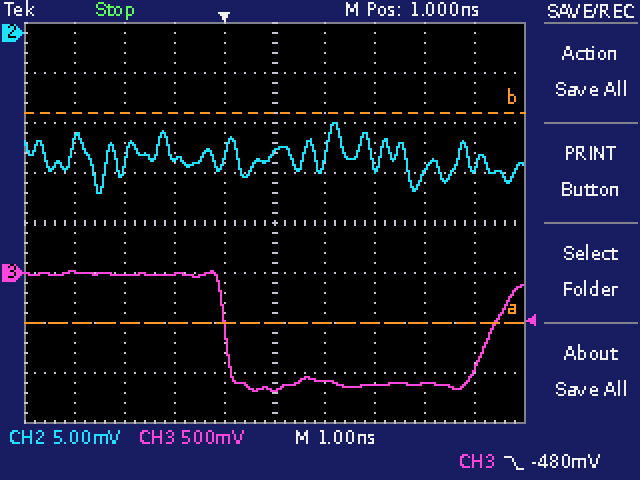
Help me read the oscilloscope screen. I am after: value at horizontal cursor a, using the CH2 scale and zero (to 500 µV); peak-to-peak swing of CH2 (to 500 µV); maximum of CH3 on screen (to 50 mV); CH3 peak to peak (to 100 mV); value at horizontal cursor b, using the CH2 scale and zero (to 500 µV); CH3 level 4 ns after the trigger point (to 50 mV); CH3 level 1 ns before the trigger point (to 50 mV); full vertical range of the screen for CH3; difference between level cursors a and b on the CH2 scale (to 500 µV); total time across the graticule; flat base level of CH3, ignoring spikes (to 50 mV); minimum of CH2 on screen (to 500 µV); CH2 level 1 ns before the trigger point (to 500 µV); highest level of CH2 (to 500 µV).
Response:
-29.0 mV
7.0 mV
0 mV
1.20 V
-8.0 mV
-1.10 V
0 mV
4 V
21.0 mV
10 ns
-1.10 V
-16.0 mV
-12.5 mV
-9.0 mV
